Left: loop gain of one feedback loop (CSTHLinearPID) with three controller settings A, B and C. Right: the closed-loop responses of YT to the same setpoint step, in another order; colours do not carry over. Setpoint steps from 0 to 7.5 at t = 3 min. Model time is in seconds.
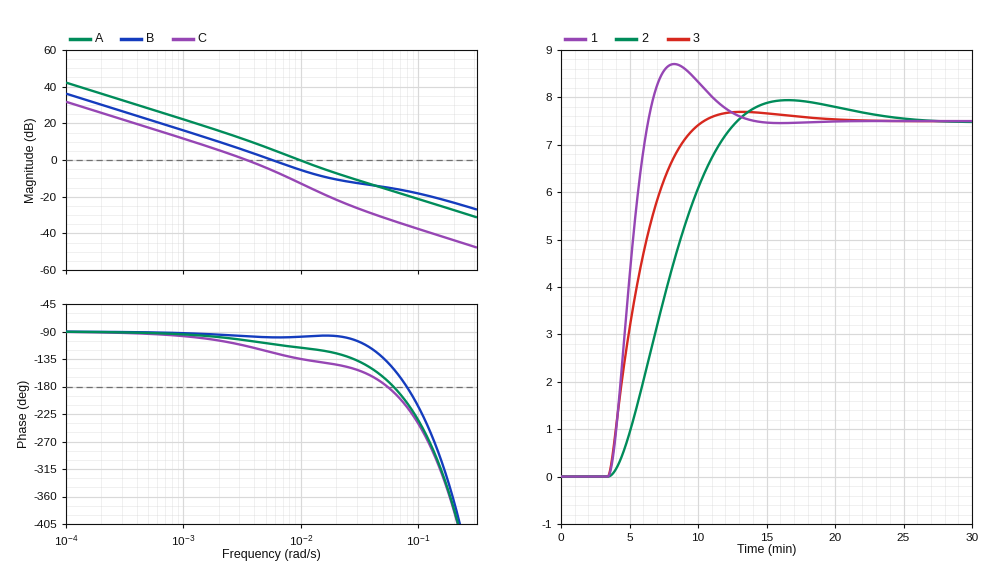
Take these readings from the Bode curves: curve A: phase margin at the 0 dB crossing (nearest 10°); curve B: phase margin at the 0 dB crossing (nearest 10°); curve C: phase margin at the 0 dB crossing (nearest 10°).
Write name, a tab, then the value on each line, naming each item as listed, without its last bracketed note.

curve A: phase margin at the 0 dB crossing	60°
curve B: phase margin at the 0 dB crossing	80°
curve C: phase margin at the 0 dB crossing	70°
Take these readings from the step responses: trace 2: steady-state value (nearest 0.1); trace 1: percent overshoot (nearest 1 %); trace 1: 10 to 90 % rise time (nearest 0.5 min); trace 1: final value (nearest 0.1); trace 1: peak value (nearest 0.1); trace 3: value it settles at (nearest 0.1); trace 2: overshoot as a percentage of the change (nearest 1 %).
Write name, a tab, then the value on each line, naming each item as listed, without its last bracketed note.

trace 2: steady-state value	7.5
trace 1: percent overshoot	16 %
trace 1: 10 to 90 % rise time	2.0 min
trace 1: final value	7.5
trace 1: peak value	8.7
trace 3: value it settles at	7.5
trace 2: overshoot as a percentage of the change	6 %
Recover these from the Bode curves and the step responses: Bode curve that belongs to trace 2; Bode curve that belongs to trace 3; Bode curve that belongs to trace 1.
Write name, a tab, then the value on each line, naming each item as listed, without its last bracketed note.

Bode curve that belongs to trace 2	C
Bode curve that belongs to trace 3	B
Bode curve that belongs to trace 1	A
